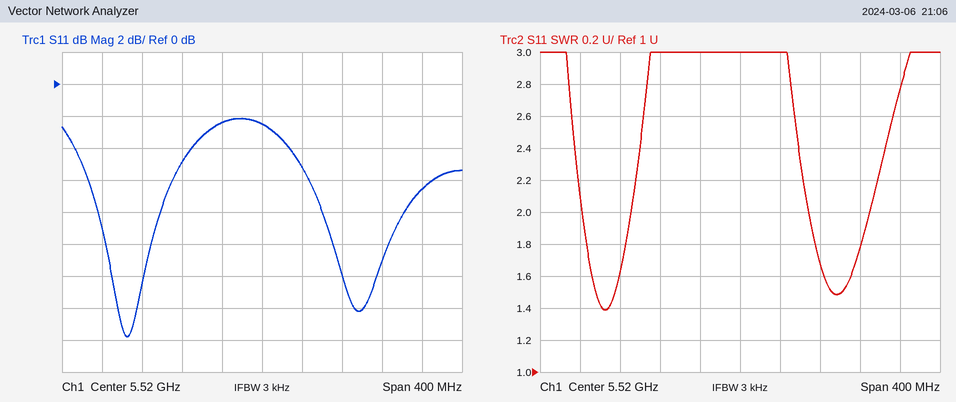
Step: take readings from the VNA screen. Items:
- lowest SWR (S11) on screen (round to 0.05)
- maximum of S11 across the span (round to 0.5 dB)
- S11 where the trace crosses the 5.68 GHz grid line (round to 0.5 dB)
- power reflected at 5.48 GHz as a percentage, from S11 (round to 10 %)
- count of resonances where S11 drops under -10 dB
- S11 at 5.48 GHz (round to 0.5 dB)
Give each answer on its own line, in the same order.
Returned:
1.40
-2.0 dB
-6.5 dB
60 %
2
-2.5 dB
